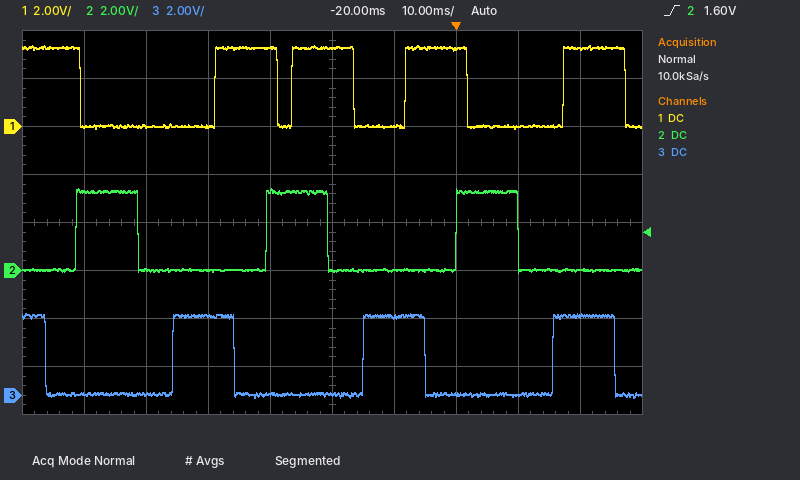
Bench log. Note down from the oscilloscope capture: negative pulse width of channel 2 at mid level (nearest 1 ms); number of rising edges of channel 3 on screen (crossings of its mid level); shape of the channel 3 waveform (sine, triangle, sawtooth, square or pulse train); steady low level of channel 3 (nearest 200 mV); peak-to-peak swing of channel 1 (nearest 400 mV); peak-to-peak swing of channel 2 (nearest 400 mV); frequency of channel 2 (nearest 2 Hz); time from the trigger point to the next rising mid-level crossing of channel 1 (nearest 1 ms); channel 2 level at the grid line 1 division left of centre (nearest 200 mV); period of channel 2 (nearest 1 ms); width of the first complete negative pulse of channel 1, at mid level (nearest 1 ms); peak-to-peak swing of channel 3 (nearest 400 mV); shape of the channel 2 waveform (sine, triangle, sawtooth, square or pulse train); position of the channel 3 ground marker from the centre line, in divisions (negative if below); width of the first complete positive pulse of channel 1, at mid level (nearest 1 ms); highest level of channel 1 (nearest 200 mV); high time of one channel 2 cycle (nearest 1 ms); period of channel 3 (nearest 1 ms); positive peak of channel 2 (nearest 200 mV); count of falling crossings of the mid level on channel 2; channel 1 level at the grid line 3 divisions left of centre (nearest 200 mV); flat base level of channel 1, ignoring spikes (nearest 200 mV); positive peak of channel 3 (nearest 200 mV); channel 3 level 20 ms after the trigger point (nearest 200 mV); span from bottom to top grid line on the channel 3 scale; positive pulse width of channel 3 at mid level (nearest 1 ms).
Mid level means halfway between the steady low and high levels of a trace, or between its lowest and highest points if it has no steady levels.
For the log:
21 ms
3
pulse train
0.0 V
3.6 V
3.6 V
32 Hz
17 ms
3.4 V
31 ms
22 ms
3.6 V
pulse train
-3.6 div
10 ms
3.4 V
10 ms
31 ms
3.4 V
3
0.0 V
0.0 V
3.4 V
3.4 V
16 V
10 ms
